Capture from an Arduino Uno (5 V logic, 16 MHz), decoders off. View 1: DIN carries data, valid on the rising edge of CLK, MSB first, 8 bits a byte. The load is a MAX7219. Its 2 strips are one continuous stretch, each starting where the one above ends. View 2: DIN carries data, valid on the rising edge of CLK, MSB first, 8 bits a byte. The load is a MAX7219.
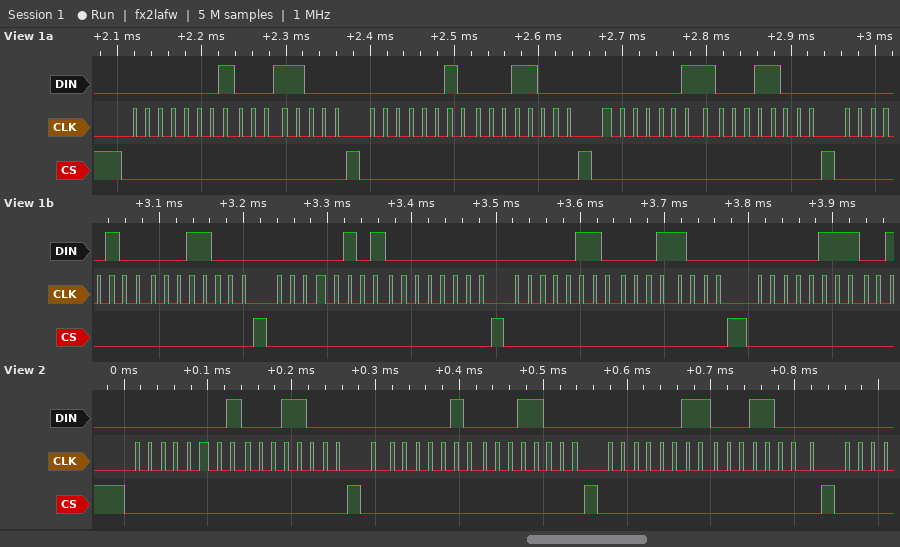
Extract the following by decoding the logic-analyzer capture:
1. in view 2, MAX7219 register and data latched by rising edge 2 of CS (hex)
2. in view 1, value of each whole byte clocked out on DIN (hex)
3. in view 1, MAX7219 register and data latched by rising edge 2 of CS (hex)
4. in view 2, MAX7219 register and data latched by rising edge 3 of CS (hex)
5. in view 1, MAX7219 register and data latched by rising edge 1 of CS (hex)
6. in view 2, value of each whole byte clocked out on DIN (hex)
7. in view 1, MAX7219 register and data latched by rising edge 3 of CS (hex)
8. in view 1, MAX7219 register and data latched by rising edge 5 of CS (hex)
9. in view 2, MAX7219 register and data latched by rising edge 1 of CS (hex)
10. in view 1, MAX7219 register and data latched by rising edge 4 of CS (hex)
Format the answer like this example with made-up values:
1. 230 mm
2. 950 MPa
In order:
1. register 0x2, data 0x18
2. 0x01 0x18 0x02 0x18 0x03 0x18 0x04 0x18 0x05 0x00 0x06 0x18 0x07
3. register 0x2, data 0x18
4. register 0x3, data 0x18
5. register 0x1, data 0x18
6. 01 18 02 18 03 18
7. register 0x3, data 0x18
8. register 0x5, data 0x00
9. register 0x1, data 0x18
10. register 0x4, data 0x18
